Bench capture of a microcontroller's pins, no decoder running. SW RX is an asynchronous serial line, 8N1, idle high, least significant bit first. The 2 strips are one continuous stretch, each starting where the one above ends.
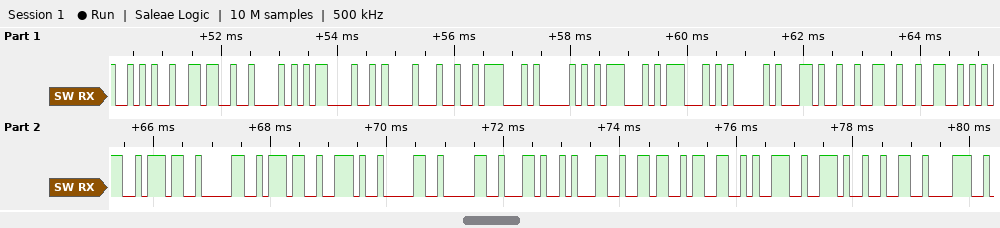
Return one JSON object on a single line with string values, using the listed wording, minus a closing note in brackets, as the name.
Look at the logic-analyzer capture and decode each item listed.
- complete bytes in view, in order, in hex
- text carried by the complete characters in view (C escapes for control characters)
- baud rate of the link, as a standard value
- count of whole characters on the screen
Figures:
{"complete bytes in view, in order, in hex": "0x2A 0x36 0x42 0x0D 0x0A 0x24 0x47 0x50 0x47 0x47 0x41 0x2C 0x32 0x32 0x35 0x37 0x30 0x37 0x2E 0x30 0x30 0x2C 0x31 0x36 0x33 0x39 0x2E 0x32 0x38", "text carried by the complete characters in view": "\"*6B\\r\\n$GPGGA,225707.00,1639.28\"", "baud rate of the link, as a standard value": "9600 baud", "count of whole characters on the screen": "29"}
